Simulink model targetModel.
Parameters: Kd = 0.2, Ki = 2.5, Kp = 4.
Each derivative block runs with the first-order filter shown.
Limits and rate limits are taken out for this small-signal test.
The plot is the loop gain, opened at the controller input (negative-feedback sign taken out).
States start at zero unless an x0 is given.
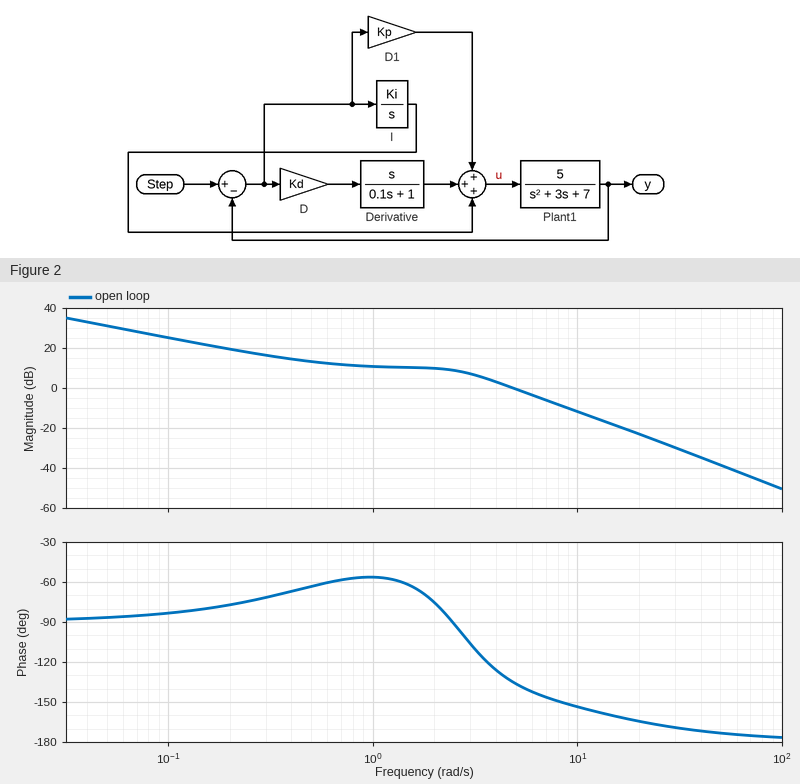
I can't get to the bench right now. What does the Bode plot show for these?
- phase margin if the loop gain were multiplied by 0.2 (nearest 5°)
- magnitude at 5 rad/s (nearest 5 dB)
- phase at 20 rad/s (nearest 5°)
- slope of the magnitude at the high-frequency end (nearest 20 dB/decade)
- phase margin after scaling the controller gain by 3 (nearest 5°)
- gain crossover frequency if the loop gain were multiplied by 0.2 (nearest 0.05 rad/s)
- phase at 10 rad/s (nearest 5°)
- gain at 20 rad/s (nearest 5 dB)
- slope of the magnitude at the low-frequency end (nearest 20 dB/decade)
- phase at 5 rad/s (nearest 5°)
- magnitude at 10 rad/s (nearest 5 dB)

115°
0 dB
-165°
-40 dB/decade
30°
0.45 rad/s
-155°
-25 dB
-20 dB/decade
-135°
-10 dB
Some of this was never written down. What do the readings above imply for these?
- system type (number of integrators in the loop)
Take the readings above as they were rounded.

1
